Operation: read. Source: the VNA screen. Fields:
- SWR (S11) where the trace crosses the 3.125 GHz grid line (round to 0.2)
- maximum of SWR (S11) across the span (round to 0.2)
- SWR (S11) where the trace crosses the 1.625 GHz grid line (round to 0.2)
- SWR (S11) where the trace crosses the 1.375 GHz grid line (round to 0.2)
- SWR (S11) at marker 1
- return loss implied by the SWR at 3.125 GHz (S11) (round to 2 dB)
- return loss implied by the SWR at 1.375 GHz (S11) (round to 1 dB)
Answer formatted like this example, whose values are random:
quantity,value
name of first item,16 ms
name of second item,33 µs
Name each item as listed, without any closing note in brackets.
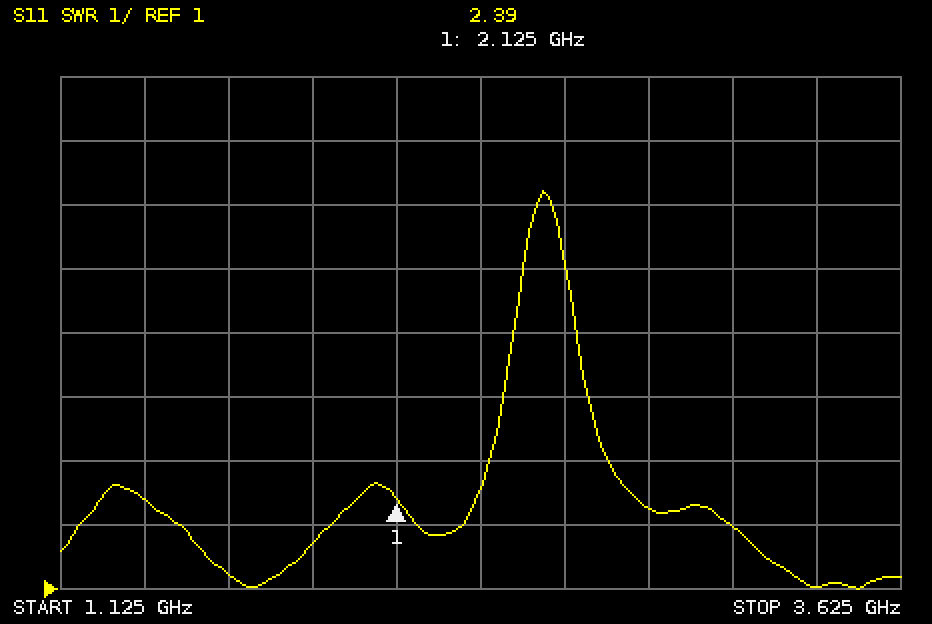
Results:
quantity,value
SWR (S11) where the trace crosses the 3.125 GHz grid line,2.0
maximum of SWR (S11) across the span,7.2
SWR (S11) where the trace crosses the 1.625 GHz grid line,1.2
SWR (S11) where the trace crosses the 1.375 GHz grid line,2.4
SWR (S11) at marker 1,2.39
return loss implied by the SWR at 3.125 GHz (S11),10 dB
return loss implied by the SWR at 1.375 GHz (S11),8 dB
